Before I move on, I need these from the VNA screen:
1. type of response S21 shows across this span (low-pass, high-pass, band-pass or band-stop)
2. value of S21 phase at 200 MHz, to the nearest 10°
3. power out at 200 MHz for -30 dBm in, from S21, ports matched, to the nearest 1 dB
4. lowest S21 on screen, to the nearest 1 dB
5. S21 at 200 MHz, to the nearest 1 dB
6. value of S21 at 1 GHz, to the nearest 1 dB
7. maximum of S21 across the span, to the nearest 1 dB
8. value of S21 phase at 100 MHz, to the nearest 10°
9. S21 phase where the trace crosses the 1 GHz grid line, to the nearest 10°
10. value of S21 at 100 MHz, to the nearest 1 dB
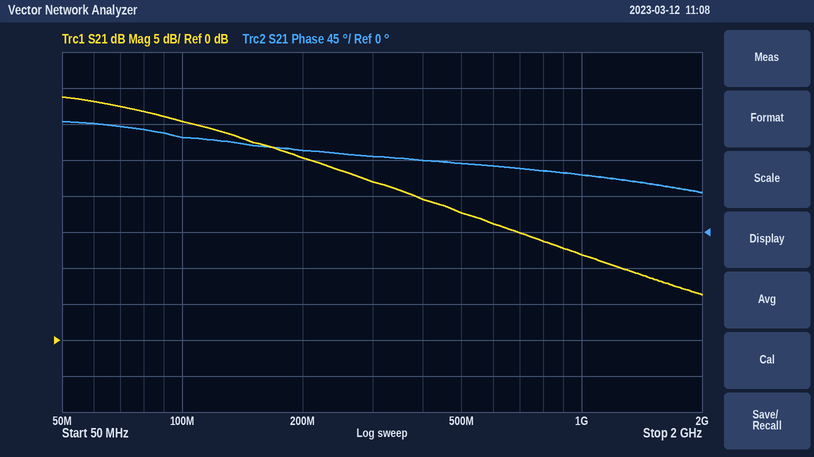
low-pass
100°
-5 dBm
6 dB
25 dB
12 dB
34 dB
120°
70°
30 dB
